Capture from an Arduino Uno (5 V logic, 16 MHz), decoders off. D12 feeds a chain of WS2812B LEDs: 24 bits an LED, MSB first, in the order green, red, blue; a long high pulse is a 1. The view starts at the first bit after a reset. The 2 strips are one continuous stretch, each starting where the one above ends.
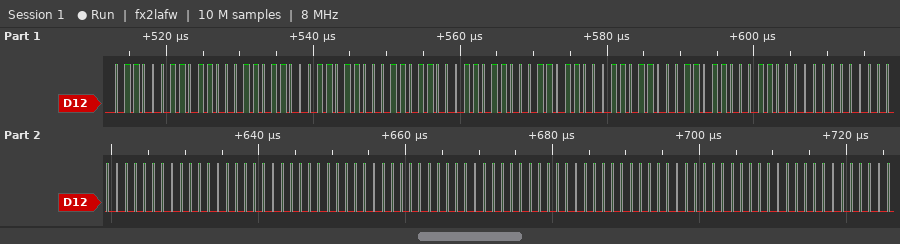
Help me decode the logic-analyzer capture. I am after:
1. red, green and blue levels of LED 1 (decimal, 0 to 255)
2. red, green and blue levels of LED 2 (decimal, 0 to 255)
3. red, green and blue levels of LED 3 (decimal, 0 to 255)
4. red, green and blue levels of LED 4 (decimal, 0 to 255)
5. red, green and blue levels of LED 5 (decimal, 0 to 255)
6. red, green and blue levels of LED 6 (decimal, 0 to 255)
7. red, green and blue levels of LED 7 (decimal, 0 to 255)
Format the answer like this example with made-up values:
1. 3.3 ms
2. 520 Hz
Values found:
1. 99, 99, 99
2. 99, 99, 99
3. 99, 99, 99
4. 0, 0, 0
5. 0, 0, 0
6. 0, 0, 0
7. 0, 0, 0
